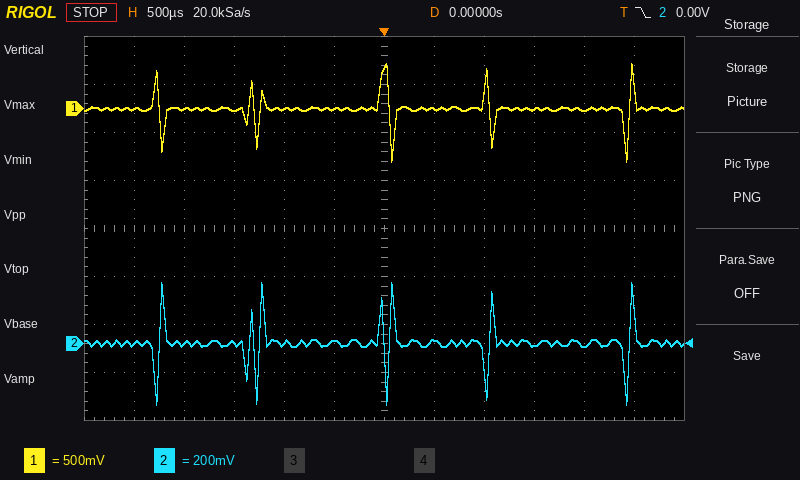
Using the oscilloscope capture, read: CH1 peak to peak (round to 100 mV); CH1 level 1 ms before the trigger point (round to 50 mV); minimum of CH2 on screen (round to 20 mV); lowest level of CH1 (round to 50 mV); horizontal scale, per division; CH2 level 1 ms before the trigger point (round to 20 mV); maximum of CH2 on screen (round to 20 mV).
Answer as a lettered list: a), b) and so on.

a) 1.00 V
b) 0 mV
c) -260 mV
d) -550 mV
e) 500 µs
f) 0 mV
g) 260 mV
